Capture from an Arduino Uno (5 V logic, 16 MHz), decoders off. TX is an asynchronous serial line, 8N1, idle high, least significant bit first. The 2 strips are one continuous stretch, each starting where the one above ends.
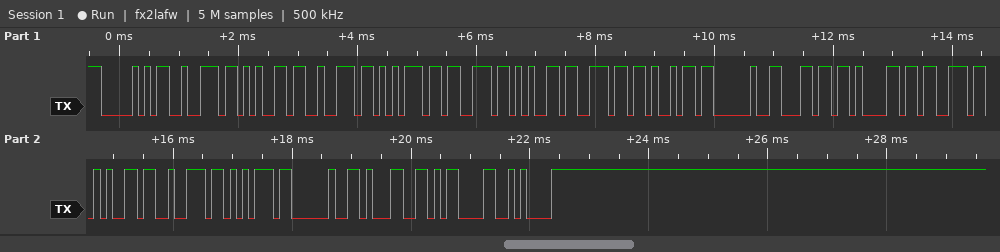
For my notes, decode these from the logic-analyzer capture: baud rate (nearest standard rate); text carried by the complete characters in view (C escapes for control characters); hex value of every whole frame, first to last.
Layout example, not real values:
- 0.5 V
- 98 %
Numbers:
- 9600 baud
- "Preruseni laseru 1\r\n"
- 0x50 0x72 0x65 0x72 0x75 0x73 0x65 0x6E 0x69 0x20 0x6C 0x61 0x73 0x65 0x72 0x75 0x20 0x31 0x0D 0x0A
